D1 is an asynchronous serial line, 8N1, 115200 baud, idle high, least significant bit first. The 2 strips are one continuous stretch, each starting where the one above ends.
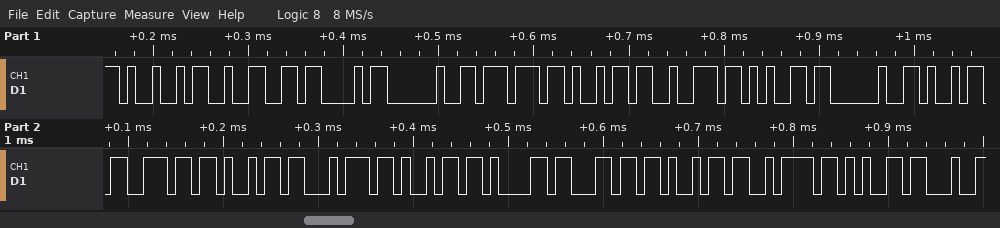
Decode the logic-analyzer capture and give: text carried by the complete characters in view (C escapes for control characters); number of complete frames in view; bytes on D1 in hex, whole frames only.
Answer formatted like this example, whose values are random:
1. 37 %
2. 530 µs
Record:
1. "I2C wire initialize"
2. 19
3. 49 32 43 20 77 69 72 65 20 69 6E 69 74 69 61 6C 69 7A 65
